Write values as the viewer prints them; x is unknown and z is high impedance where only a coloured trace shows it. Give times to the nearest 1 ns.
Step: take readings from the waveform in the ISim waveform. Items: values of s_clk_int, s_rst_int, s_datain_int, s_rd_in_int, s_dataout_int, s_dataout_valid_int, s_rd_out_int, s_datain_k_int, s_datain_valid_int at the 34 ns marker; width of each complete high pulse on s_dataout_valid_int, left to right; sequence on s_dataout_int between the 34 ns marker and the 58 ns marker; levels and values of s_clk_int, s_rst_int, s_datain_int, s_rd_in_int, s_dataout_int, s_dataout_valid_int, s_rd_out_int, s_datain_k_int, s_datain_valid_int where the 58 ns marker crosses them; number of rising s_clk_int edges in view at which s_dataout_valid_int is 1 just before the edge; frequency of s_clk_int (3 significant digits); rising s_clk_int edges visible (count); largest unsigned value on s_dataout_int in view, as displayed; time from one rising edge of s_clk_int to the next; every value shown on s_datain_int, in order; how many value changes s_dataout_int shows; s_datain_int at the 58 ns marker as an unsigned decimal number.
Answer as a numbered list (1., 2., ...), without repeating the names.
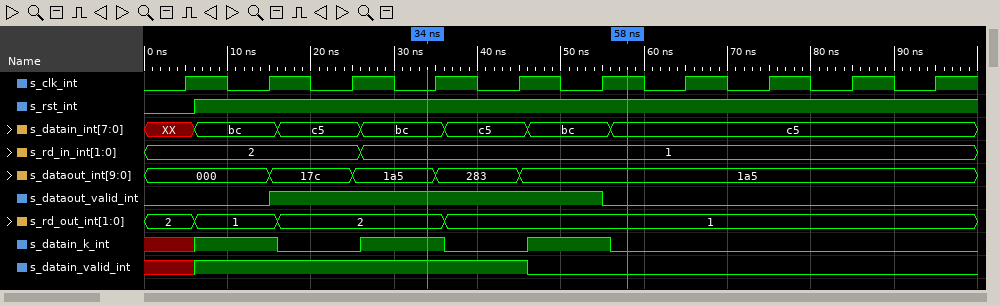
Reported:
1. s_clk_int=0, s_rst_int=1, s_datain_int=bc, s_rd_in_int=1, s_dataout_int=1a5, s_dataout_valid_int=1, s_rd_out_int=2, s_datain_k_int=1, s_datain_valid_int=1
2. 40 ns
3. 1a5, 283, 1a5
4. s_clk_int=1, s_rst_int=1, s_datain_int=c5, s_rd_in_int=1, s_dataout_int=1a5, s_dataout_valid_int=0, s_rd_out_int=1, s_datain_k_int=0, s_datain_valid_int=0
5. 4
6. 100 MHz
7. 10
8. 283
9. 10 ns
10. XX, bc, c5, bc, c5, bc, c5
11. 4
12. 197
